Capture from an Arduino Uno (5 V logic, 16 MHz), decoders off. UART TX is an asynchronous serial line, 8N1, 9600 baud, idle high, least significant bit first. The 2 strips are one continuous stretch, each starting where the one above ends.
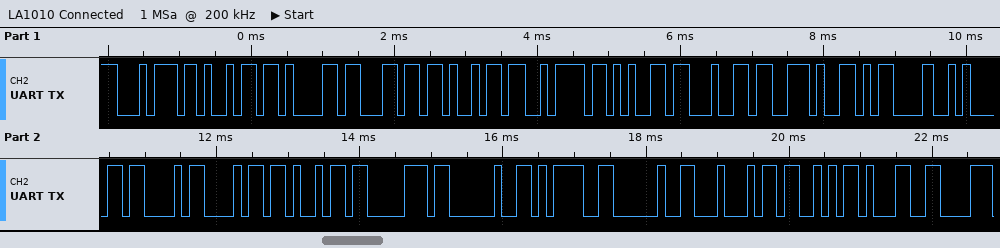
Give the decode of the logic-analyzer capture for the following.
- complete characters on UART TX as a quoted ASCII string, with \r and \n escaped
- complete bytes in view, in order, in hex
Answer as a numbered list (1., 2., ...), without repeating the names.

1. "tialized.\r\nChip = DS1"
2. 74 69 61 6C 69 7A 65 64 2E 0D 0A 43 68 69 70 20 3D 20 44 53 31
